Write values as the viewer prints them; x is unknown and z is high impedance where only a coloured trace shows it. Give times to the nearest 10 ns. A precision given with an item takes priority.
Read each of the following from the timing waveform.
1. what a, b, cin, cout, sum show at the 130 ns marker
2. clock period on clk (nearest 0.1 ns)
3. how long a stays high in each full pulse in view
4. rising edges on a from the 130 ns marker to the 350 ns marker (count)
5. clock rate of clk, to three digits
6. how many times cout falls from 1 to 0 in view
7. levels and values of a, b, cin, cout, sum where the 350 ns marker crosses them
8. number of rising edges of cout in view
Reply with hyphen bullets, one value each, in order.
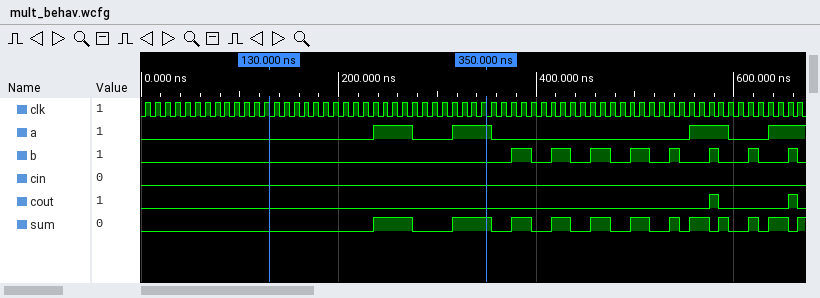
- a=0, b=0, cin=0, cout=0, sum=0
- 10 ns
- 40 ns, 40 ns, 40 ns
- 2
- 100 MHz
- 2
- a=1, b=0, cin=0, cout=0, sum=1
- 2
